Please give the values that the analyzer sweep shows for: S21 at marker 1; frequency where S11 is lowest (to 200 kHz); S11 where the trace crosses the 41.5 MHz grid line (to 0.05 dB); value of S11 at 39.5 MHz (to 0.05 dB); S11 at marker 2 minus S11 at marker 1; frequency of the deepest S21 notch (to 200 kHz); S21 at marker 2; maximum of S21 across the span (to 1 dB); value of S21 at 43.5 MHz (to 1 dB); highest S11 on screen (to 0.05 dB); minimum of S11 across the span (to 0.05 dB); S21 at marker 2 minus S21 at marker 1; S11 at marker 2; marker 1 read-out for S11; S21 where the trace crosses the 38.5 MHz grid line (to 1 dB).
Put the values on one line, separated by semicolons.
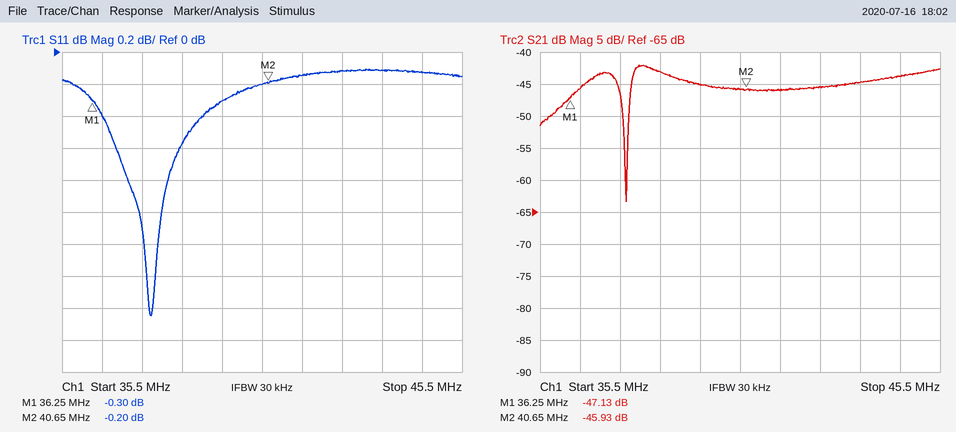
-47.13 dB; 37.8 MHz; -0.15 dB; -0.30 dB; 0.10 dB; 37.6 MHz; -45.93 dB; -42 dB; -45 dB; -0.10 dB; -1.65 dB; 1.20 dB; -0.20 dB; -0.30 dB; -43 dB
